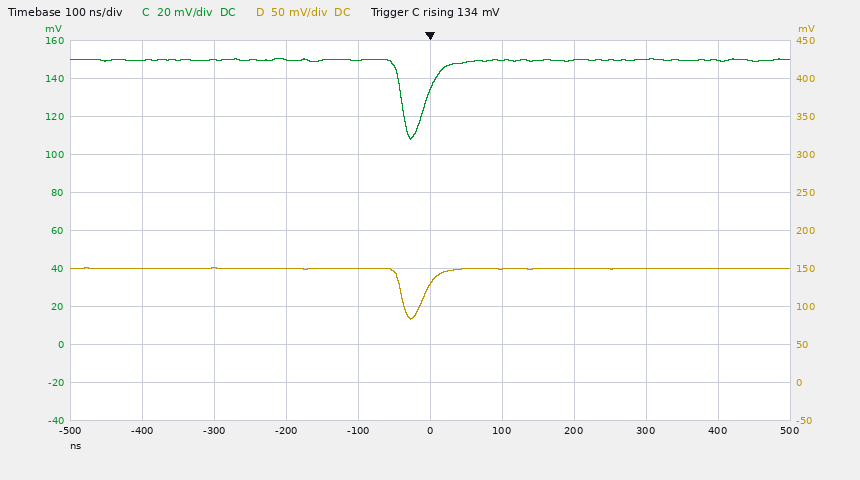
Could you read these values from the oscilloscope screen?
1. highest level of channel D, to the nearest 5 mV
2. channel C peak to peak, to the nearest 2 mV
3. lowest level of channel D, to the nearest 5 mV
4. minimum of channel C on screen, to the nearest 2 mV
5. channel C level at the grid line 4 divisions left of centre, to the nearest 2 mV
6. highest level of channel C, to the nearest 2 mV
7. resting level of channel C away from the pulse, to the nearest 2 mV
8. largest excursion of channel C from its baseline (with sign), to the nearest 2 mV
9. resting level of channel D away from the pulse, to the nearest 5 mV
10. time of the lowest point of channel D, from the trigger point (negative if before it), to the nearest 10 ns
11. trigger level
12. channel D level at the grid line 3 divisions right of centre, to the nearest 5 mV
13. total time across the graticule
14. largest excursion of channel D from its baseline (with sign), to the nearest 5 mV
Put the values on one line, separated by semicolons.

150 mV; 42 mV; 85 mV; 108 mV; 150 mV; 150 mV; 150 mV; -42 mV; 150 mV; -30 ns; 134 mV; 150 mV; 1 µs; -65 mV
